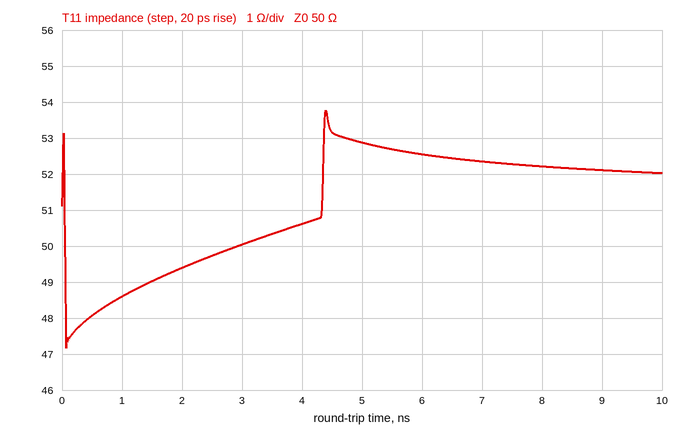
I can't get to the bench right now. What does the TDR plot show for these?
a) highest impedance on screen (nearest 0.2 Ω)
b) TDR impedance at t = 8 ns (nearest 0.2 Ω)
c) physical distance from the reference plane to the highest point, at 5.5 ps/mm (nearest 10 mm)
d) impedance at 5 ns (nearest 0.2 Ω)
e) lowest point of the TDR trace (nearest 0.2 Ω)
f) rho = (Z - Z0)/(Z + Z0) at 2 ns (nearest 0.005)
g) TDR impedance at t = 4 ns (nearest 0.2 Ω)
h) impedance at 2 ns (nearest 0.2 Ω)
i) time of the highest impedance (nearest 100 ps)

53.8 Ω
52.2 Ω
400 mm
52.8 Ω
47.2 Ω
-0.005
50.6 Ω
49.4 Ω
4.4 ns
